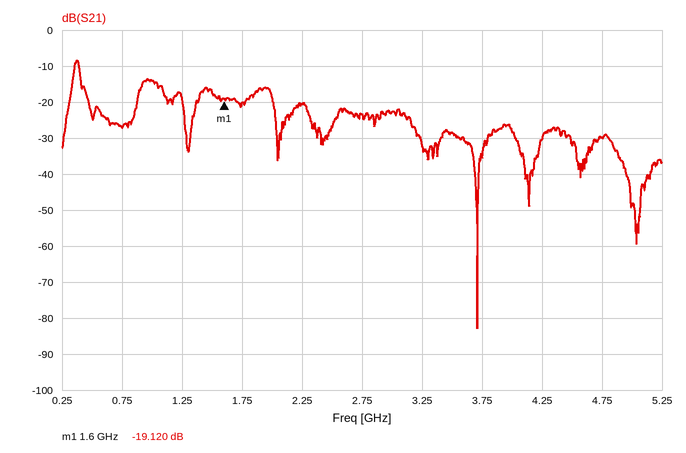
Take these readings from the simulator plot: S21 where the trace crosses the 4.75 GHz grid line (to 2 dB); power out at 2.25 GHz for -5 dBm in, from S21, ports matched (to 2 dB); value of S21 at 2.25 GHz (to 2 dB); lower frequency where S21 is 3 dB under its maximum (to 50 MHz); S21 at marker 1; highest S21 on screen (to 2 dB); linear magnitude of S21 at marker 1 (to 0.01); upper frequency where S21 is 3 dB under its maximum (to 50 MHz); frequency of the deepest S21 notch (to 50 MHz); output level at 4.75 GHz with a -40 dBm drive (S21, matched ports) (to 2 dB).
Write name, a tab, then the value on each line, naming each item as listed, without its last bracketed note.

S21 where the trace crosses the 4.75 GHz grid line	-30 dB
power out at 2.25 GHz for -5 dBm in, from S21, ports matched	-26 dBm
value of S21 at 2.25 GHz	-20 dB
lower frequency where S21 is 3 dB under its maximum	350 MHz
S21 at marker 1	-19.120 dB
highest S21 on screen	-8 dB
linear magnitude of S21 at marker 1	0.11
upper frequency where S21 is 3 dB under its maximum	400 MHz
frequency of the deepest S21 notch	3.70 GHz
output level at 4.75 GHz with a -40 dBm drive (S21, matched ports)	-70 dBm
